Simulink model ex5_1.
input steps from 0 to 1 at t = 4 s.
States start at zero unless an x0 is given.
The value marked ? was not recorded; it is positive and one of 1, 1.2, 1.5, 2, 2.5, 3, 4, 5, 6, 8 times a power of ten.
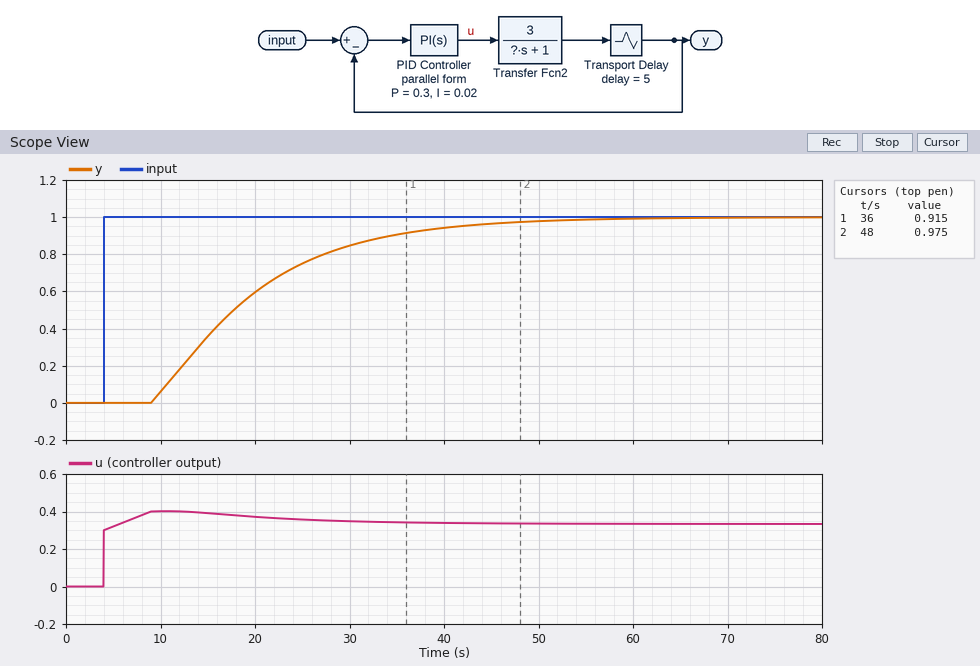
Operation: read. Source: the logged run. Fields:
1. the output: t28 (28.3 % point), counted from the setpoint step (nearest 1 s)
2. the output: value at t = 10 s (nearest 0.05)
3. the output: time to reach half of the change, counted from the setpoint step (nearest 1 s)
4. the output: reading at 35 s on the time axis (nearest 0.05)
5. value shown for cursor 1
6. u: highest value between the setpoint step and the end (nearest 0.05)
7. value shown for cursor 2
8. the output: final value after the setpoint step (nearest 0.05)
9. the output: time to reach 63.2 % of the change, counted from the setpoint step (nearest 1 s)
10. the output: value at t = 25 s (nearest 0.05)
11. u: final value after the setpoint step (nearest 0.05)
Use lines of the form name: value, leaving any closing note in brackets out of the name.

the output: t28 (28.3 % point), counted from the setpoint step: 10 s
the output: value at t = 10 s: 0.05
the output: time to reach half of the change, counted from the setpoint step: 14 s
the output: reading at 35 s on the time axis: 0.90
value shown for cursor 1: 0.915
u: highest value between the setpoint step and the end: 0.40
value shown for cursor 2: 0.975
the output: final value after the setpoint step: 1.00
the output: time to reach 63.2 % of the change, counted from the setpoint step: 17 s
the output: value at t = 25 s: 0.75
u: final value after the setpoint step: 0.35
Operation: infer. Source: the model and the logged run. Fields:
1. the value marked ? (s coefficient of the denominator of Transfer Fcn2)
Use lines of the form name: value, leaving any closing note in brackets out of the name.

the value marked ?: 15
